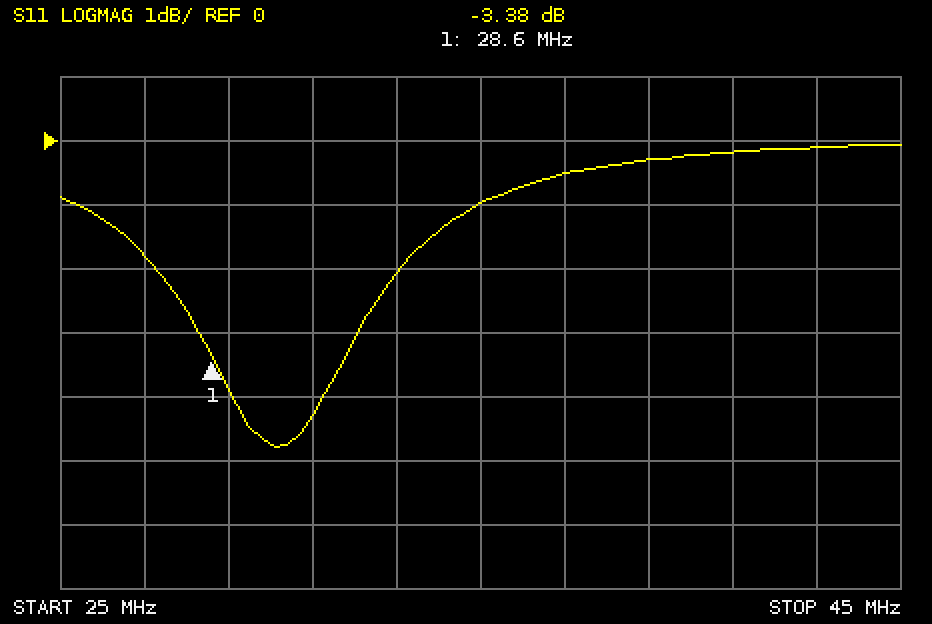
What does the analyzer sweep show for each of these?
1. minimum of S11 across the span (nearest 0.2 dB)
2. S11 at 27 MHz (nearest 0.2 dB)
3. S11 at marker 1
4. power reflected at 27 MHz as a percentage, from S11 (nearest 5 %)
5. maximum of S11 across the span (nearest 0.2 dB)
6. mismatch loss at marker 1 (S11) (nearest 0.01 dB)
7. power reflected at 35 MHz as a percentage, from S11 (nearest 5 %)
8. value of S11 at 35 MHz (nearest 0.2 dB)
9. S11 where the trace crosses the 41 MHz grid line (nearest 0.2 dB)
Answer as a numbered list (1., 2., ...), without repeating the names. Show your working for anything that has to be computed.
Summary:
1. -4.8 dB
2. -1.8 dB
3. -3.38 dB
4. 10^(-1.8/10) ≈ 66.1 %, so 65 % to the nearest 5 %
5. 0.0 dB
6. −10 log10(1 − 10^(-3.38/10)) ≈ 2.67 dB
7. 10^(-1/10) ≈ 79.4 %, so 80 % to the nearest 5 %
8. -1.0 dB
9. -0.2 dB
